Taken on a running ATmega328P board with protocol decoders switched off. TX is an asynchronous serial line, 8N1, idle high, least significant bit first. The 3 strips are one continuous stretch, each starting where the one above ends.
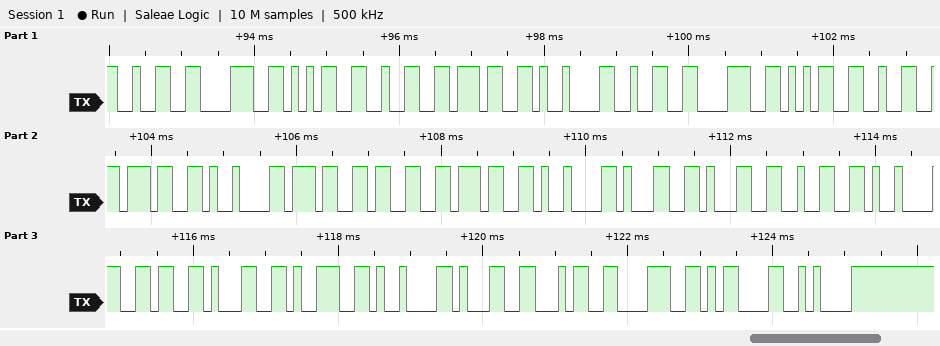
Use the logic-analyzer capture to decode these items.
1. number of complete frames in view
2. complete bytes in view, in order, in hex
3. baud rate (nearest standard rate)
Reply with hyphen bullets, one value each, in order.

- 29
- 32 38 35 32 37 09 32 38 35 32 37 09 37 33 37 09 31 31 32 09 36 31 39 09 31 34 38 0D 0A
- 9600 baud
